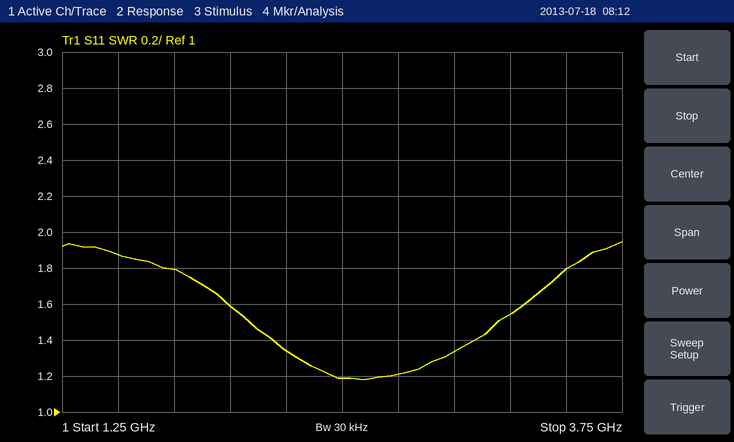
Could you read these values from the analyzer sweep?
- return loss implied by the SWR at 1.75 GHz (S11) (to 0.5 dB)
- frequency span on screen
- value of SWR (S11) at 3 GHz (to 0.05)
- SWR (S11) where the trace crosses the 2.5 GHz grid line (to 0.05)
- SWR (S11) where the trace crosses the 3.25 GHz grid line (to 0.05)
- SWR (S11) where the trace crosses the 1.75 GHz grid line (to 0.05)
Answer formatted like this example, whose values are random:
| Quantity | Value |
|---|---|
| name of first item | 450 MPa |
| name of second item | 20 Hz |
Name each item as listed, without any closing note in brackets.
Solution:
| Quantity | Value |
|---|---|
| return loss implied by the SWR at 1.75 GHz (S11) | 11.0 dB |
| frequency span on screen | 2.5 GHz |
| value of SWR (S11) at 3 GHz | 1.35 |
| SWR (S11) where the trace crosses the 2.5 GHz grid line | 1.20 |
| SWR (S11) where the trace crosses the 3.25 GHz grid line | 1.55 |
| SWR (S11) where the trace crosses the 1.75 GHz grid line | 1.80 |
